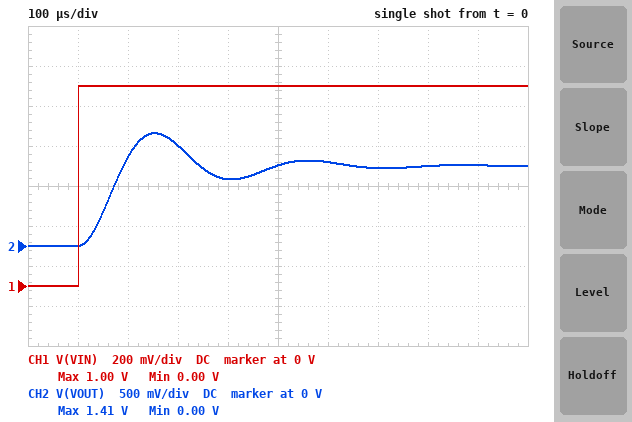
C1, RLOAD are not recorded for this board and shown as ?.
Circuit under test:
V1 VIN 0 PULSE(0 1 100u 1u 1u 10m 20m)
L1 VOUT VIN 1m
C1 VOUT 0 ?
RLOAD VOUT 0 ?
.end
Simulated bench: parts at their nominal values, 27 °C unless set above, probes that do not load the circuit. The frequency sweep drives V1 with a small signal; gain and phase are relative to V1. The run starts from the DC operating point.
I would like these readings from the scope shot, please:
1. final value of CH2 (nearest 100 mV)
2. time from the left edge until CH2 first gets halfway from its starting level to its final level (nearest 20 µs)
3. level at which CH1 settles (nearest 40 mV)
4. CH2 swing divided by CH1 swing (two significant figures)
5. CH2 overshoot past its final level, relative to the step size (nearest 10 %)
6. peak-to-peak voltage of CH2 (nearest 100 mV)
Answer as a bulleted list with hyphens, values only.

- 1.0 V
- 160 µs
- 1.00 V
- 1.4
- 40 %
- 1.4 V
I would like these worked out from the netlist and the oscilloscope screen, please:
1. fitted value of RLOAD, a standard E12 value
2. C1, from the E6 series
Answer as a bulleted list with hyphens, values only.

- 39 Ω
- 2.2 µF
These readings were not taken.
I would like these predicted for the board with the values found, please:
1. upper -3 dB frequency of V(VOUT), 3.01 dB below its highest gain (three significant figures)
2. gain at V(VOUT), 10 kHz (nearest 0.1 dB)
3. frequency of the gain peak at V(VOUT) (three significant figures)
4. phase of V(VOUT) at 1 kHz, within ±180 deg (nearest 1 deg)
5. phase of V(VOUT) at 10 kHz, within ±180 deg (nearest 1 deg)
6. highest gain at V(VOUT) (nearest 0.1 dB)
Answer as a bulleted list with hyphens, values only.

- 3.98 kHz
- -17.9 dB
- 3.13 kHz
- -10 deg
- -168 deg
- 5.6 dB
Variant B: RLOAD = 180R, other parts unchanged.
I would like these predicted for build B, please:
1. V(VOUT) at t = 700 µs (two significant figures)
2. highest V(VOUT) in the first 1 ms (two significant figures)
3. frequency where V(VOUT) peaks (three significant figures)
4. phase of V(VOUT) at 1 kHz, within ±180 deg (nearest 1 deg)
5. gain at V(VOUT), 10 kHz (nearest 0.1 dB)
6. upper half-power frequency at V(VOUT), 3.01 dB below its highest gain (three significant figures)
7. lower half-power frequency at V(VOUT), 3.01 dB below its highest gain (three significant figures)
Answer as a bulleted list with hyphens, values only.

- 530 mV
- 1.8 V
- 3.38 kHz
- -2 deg
- -17.7 dB
- 3.58 kHz
- 3.17 kHz
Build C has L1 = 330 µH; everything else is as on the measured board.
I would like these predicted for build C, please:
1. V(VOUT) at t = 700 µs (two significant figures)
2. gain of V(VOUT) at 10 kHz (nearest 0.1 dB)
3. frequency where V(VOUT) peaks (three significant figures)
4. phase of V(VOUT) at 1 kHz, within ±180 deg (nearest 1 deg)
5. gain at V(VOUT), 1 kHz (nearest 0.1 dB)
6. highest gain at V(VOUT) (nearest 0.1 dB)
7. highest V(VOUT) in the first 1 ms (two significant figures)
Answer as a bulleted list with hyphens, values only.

- 1.0 V
- -5.8 dB
- 5.76 kHz
- -3 deg
- 0.2 dB
- 10.2 dB
- 1.6 V
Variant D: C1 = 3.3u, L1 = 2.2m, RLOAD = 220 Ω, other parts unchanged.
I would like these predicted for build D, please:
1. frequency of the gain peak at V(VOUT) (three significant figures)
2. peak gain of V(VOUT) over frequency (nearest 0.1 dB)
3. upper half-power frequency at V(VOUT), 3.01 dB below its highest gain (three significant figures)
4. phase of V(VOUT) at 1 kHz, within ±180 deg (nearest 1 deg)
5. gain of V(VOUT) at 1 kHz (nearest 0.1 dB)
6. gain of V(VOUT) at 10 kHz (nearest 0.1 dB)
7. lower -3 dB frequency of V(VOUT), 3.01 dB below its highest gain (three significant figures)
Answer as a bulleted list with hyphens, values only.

- 1.86 kHz
- 18.6 dB
- 1.97 kHz
- -5 deg
- 2.9 dB
- -28.8 dB
- 1.75 kHz
